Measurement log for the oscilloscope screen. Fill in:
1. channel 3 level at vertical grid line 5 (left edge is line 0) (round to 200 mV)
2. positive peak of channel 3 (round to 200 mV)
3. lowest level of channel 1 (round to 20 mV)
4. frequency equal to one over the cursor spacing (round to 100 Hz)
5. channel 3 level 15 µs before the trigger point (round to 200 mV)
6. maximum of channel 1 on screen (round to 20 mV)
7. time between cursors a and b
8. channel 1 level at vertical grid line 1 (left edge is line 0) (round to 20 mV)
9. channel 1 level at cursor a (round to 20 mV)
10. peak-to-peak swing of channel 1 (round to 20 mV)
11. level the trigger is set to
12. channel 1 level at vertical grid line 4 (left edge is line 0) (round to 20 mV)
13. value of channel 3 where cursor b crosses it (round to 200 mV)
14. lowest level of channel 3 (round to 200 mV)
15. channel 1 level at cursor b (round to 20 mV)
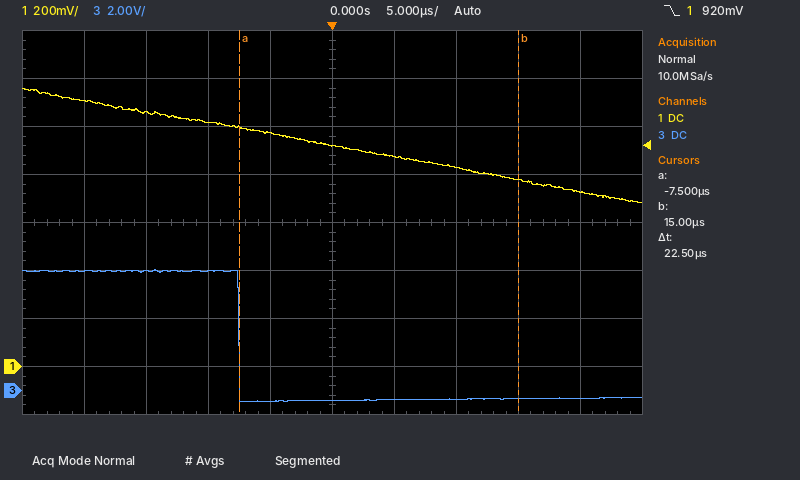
-400 mV
5.0 V
680 mV
44.4 kHz
5.0 V
1.16 V
22.5 µs
1.10 V
1.00 V
480 mV
920 mV
980 mV
-400 mV
-400 mV
780 mV
